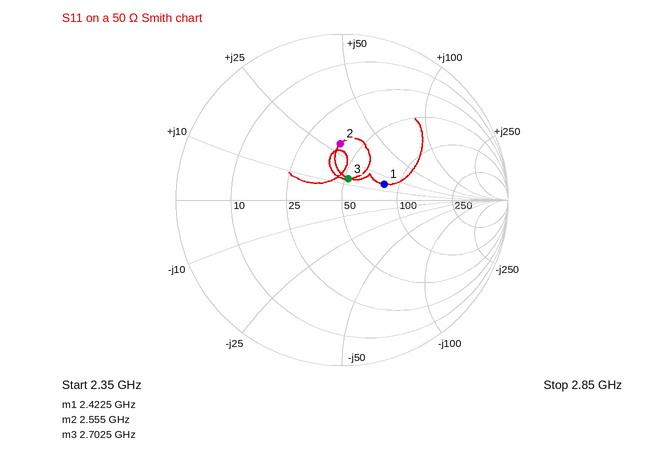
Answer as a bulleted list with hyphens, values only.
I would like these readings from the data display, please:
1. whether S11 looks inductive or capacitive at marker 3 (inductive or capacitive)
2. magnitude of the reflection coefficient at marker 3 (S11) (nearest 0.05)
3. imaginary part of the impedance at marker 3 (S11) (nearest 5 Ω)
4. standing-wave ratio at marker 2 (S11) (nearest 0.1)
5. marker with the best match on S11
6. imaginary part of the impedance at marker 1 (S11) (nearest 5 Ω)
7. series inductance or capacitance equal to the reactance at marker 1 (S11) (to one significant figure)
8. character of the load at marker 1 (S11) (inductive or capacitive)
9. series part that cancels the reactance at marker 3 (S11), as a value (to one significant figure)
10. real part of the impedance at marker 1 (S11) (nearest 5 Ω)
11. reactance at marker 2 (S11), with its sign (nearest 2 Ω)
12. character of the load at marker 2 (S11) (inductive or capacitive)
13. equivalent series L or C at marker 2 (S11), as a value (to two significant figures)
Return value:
- inductive
- 0.15
- +15 Ω
- 2.0
- marker 3
- +15 Ω
- 1 nH
- inductive
- 4 pF
- 80 Ω
- +30 Ω
- inductive
- 1.9 nH
